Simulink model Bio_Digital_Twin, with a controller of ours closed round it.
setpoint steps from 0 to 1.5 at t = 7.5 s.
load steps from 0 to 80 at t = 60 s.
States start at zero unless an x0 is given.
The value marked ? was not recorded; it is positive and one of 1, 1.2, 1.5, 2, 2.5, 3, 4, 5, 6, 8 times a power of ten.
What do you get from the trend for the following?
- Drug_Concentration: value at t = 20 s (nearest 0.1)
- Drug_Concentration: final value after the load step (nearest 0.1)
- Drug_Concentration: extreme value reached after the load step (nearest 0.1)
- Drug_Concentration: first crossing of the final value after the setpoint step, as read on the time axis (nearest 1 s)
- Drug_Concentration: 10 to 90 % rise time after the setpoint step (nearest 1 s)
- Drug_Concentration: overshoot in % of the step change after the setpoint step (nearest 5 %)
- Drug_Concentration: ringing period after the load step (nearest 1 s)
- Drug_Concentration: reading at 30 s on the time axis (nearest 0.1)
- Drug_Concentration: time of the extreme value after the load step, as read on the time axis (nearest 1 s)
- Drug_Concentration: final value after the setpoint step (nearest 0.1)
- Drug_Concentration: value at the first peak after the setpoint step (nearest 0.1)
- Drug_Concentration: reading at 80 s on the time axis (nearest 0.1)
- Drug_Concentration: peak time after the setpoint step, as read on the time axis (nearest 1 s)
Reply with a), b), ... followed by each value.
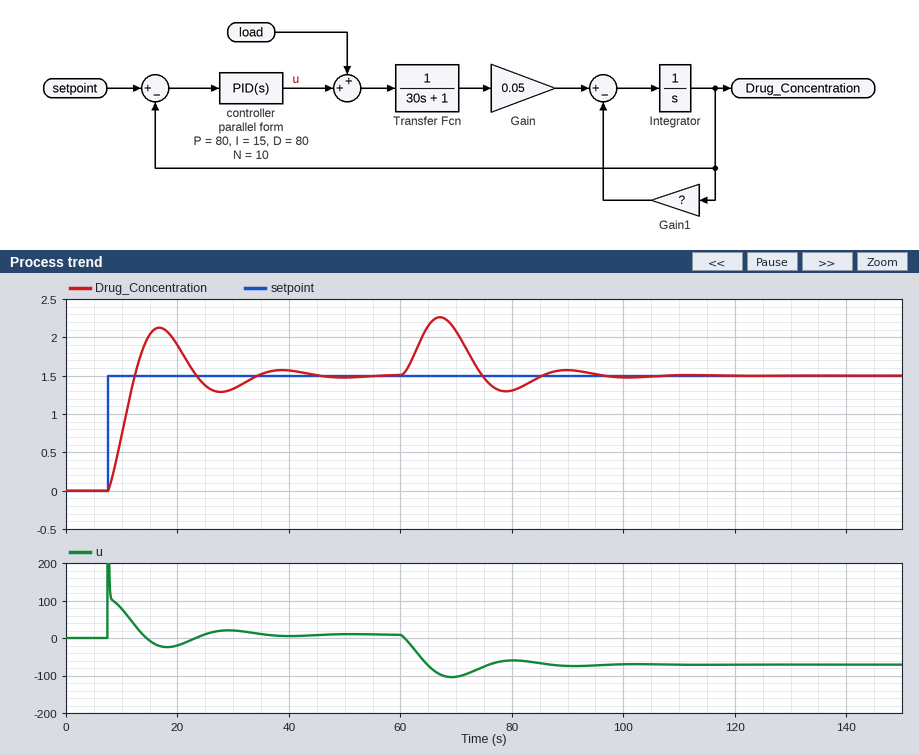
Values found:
a) 1.9
b) 1.5
c) 2.3
d) 12 s
e) 4 s
f) 40 %
g) 23 s
h) 1.3
i) 67 s
j) 1.5
k) 2.1
l) 1.3
m) 17 s
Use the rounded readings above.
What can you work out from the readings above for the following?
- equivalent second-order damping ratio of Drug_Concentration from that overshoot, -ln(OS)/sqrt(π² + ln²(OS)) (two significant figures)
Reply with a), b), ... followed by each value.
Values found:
a) 0.28
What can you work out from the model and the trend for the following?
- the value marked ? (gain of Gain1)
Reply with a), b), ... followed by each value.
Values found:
a) 0.3
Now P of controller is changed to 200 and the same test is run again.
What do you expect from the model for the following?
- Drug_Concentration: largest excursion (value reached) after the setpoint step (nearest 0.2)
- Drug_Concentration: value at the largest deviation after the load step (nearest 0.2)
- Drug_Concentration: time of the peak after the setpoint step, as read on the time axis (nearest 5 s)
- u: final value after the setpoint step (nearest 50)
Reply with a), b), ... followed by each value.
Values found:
a) 2.0
b) 2.0
c) 15 s
d) 0
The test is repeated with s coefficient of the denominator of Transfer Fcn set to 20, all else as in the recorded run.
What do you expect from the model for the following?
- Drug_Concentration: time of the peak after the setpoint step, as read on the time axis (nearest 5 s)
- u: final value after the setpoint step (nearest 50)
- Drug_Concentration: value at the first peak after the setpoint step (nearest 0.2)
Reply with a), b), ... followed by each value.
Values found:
a) 15 s
b) 0
c) 2.0
